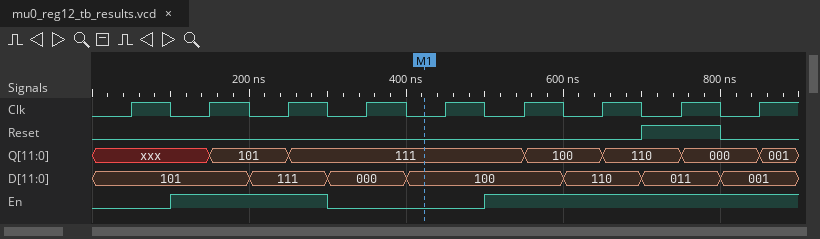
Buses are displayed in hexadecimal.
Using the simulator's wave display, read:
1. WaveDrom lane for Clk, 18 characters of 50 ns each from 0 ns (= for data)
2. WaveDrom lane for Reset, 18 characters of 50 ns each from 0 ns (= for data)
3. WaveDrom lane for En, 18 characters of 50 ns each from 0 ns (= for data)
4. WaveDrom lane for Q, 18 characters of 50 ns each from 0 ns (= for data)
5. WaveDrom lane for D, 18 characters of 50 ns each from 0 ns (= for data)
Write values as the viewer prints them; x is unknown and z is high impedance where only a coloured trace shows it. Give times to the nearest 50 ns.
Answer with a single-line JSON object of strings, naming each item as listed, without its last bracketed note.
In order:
{"WaveDrom lane for Clk, 18 characters of 50 ns each from 0 ns": "{name: 'Clk', wave: '010101010101010101'}", "WaveDrom lane for Reset, 18 characters of 50 ns each from 0 ns": "{name: 'Reset', wave: '0.............1.0.'}", "WaveDrom lane for En, 18 characters of 50 ns each from 0 ns": "{name: 'En', wave: '0.1...0...1.......'}", "WaveDrom lane for Q, 18 characters of 50 ns each from 0 ns": "{name: 'Q', wave: 'x..=.=.....=.=.=.=', data: '101 111 100 110 000 001'}", "WaveDrom lane for D, 18 characters of 50 ns each from 0 ns": "{name: 'D', wave: '=...=.=.=...=.=.=.', data: '101 111 000 100 110 011 001'}"}
